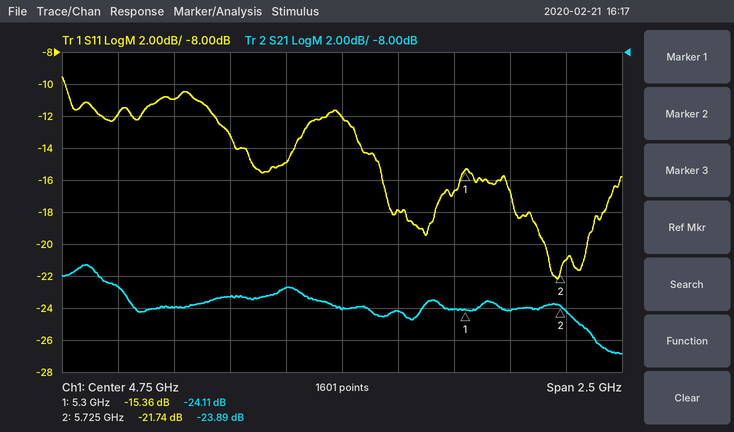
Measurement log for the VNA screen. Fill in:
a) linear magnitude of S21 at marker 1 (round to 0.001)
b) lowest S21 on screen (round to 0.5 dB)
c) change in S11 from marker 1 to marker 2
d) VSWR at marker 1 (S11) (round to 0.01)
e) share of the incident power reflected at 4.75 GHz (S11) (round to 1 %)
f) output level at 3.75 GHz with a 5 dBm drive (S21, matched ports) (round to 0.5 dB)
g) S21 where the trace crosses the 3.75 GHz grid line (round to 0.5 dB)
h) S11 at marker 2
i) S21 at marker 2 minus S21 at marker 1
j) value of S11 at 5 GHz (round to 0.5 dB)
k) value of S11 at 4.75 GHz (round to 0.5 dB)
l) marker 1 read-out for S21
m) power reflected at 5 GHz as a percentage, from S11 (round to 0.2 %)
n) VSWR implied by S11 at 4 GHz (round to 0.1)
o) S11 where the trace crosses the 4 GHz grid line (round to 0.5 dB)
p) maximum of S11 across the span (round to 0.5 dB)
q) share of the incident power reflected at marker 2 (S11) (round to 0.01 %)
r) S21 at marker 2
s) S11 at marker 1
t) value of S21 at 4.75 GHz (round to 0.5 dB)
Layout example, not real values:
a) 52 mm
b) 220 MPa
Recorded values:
a) 0.062
b) -27.0 dB
c) -6.38 dB
d) 1.41
e) 6 %
f) -17.5 dBm
g) -22.5 dB
h) -21.74 dB
i) 0.22 dB
j) -18.0 dB
k) -12.0 dB
l) -24.11 dB
m) 1.6 %
n) 1.8
o) -11.0 dB
p) -9.5 dB
q) 0.67 %
r) -23.89 dB
s) -15.36 dB
t) -24.0 dB
